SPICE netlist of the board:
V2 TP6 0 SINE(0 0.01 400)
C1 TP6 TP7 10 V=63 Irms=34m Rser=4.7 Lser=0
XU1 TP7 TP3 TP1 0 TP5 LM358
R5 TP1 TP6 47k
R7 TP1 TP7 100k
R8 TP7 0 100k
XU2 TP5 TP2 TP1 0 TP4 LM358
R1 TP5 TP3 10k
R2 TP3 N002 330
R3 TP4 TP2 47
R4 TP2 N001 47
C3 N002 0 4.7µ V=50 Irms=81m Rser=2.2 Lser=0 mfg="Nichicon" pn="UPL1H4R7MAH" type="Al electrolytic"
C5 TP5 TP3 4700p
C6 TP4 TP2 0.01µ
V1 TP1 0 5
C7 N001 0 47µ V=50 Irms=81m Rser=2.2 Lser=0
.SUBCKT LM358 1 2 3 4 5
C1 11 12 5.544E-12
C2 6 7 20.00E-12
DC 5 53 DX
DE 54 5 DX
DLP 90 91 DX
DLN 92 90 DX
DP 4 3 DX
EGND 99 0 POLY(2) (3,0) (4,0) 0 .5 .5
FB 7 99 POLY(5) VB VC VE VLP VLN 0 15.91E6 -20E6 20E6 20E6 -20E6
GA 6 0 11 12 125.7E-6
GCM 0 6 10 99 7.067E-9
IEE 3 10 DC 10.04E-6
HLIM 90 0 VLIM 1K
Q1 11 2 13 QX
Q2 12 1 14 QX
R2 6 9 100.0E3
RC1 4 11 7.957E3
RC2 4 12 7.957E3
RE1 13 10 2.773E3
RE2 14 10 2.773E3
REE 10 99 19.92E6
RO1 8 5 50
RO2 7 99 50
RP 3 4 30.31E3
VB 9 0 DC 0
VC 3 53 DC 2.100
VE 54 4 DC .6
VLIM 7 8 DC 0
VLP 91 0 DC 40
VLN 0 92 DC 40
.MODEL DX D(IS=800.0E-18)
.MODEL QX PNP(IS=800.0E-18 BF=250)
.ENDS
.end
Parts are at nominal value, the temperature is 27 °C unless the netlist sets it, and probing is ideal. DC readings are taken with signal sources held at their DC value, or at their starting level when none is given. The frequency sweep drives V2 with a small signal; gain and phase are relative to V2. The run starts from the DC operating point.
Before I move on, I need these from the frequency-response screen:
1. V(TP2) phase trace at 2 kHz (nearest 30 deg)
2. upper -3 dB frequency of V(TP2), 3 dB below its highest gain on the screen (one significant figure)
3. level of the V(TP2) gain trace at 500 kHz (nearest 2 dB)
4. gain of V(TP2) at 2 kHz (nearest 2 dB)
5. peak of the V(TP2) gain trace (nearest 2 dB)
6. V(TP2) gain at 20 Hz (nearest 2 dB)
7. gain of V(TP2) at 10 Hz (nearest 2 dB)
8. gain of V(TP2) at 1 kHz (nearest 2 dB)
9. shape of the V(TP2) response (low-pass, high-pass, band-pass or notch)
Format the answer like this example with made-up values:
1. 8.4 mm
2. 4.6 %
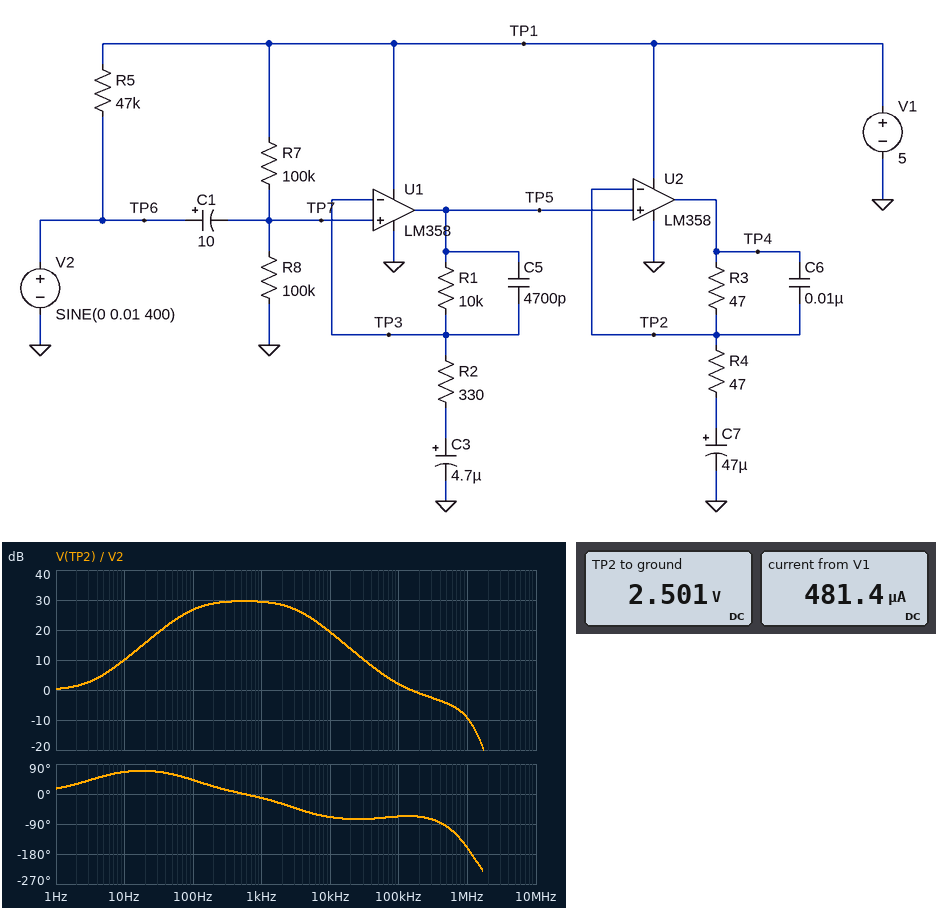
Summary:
1. -30 deg
2. 3 kHz
3. -4 dB
4. 28 dB
5. 30 dB
6. 16 dB
7. 10 dB
8. 30 dB
9. band-pass
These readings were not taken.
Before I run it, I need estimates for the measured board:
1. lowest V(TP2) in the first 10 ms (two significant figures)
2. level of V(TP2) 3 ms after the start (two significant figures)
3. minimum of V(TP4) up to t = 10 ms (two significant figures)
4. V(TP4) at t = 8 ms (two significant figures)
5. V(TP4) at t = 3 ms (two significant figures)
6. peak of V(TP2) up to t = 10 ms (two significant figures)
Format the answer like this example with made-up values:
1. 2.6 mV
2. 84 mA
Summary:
1. 2.2 V
2. 2.8 V
3. 1.9 V
4. 3.1 V
5. 3.1 V
6. 2.8 V
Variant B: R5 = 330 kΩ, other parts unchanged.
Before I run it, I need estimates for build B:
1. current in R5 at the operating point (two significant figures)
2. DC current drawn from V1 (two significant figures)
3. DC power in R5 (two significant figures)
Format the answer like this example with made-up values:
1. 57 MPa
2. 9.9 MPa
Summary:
1. 15 µA
2. 390 µA
3. 76 µW
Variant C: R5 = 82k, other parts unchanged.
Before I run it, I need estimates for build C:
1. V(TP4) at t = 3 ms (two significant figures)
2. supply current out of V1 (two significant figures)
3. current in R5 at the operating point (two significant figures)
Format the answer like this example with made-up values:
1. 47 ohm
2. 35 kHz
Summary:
1. 3.1 V
2. 440 µA
3. 61 µA
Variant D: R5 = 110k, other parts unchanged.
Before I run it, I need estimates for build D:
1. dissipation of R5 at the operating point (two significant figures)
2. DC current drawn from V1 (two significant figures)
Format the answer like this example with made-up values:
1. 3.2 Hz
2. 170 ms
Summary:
1. 230 µW
2. 420 µA
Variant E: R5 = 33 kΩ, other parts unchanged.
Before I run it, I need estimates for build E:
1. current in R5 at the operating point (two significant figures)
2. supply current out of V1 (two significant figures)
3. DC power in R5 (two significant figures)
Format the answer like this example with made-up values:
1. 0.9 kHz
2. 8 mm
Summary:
1. 150 µA
2. 530 µA
3. 760 µW
